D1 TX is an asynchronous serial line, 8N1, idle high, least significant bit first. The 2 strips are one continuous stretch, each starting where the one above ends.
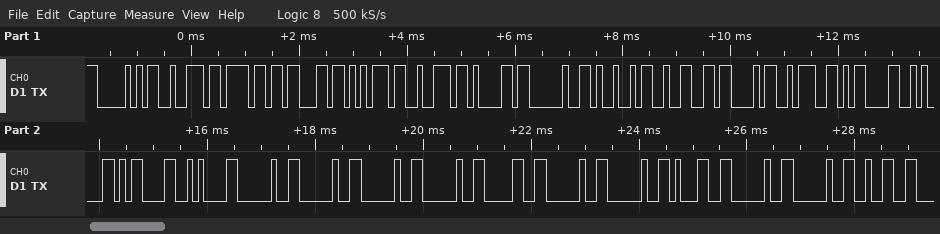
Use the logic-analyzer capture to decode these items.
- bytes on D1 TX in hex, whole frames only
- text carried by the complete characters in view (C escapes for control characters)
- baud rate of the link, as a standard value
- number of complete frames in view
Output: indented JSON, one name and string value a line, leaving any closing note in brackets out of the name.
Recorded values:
{
  "bytes on D1 TX in hex, whole frames only": "50 72 6F 63 75 72 61 20 49 32 43 3A 0D 0A 0D 0A 20 20 20 20 30 20 20 31 20 20 32",
  "text carried by the complete characters in view": "\"Procura I2C:\\r\\n\\r\\n    0  1  2\"",
  "baud rate of the link, as a standard value": "9600 baud",
  "number of complete frames in view": "27"
}
